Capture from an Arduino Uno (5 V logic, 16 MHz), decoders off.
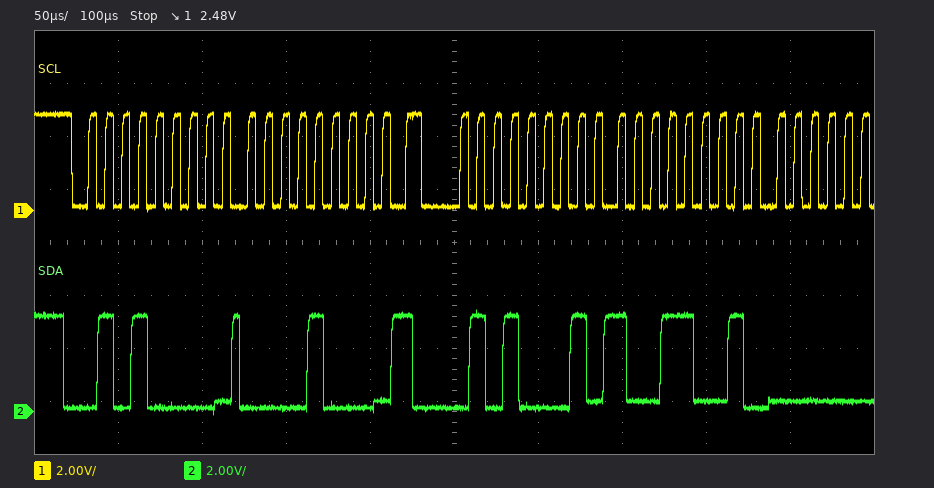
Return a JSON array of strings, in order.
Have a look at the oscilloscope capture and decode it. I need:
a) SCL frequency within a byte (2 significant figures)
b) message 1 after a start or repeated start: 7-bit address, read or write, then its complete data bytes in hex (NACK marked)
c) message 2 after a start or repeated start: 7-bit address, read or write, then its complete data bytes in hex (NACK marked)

["100 kHz", "0x28 write: 08", "0x28 read: 99"]
